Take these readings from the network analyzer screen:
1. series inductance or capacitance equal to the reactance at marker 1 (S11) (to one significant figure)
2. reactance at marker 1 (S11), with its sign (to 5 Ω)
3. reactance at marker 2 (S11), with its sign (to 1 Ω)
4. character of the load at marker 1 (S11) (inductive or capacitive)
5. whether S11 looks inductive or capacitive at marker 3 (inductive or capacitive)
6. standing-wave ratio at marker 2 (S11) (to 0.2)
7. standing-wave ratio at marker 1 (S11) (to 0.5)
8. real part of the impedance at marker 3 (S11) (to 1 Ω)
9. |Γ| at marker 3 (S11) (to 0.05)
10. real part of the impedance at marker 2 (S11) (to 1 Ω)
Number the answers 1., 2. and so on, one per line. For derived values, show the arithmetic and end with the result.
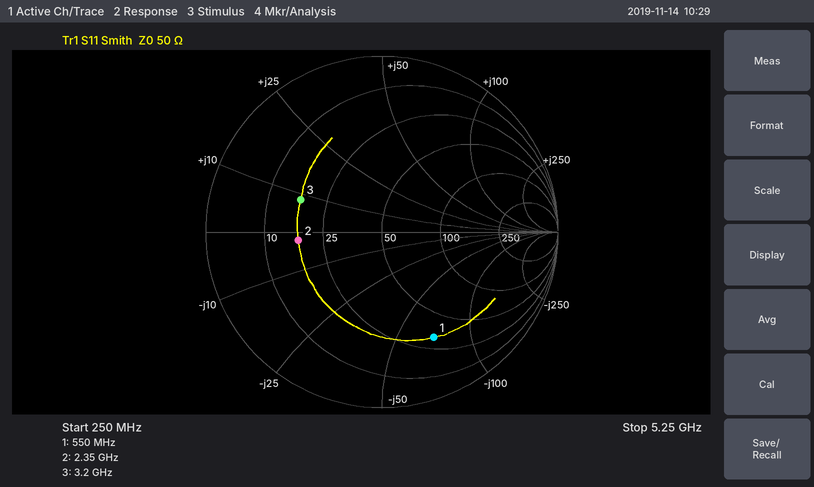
1. C = 1/(2π × 550 MHz × 70 Ω) ≈ 4 pF
2. -70 Ω
3. -2 Ω
4. capacitive
5. inductive
6. 2.8
7. 5.0
8. 17 Ω
9. 0.50
10. 18 Ω
